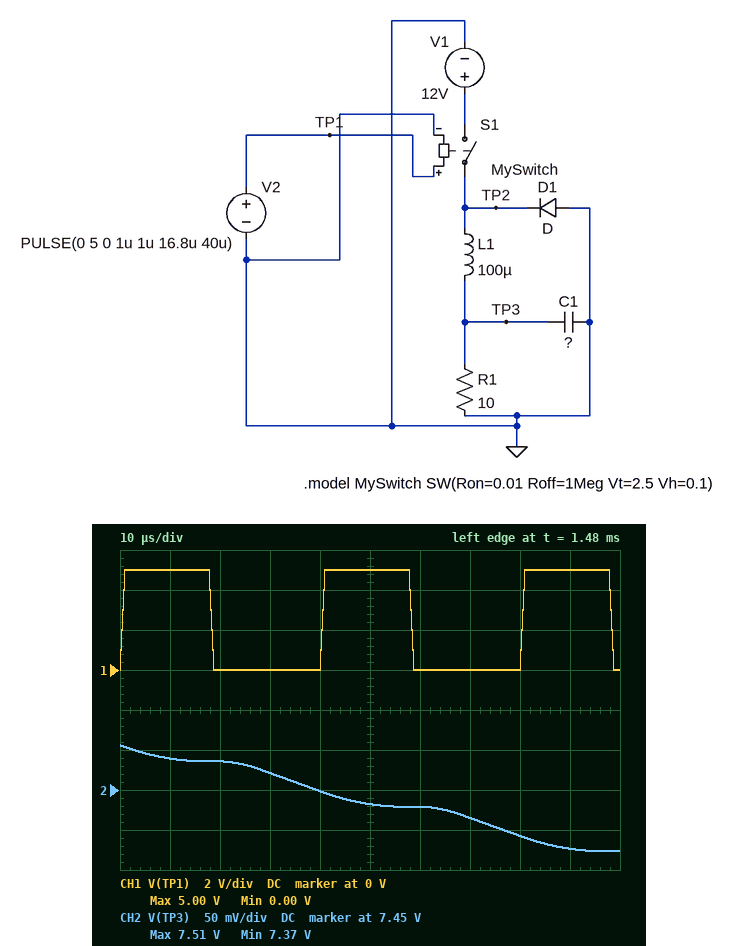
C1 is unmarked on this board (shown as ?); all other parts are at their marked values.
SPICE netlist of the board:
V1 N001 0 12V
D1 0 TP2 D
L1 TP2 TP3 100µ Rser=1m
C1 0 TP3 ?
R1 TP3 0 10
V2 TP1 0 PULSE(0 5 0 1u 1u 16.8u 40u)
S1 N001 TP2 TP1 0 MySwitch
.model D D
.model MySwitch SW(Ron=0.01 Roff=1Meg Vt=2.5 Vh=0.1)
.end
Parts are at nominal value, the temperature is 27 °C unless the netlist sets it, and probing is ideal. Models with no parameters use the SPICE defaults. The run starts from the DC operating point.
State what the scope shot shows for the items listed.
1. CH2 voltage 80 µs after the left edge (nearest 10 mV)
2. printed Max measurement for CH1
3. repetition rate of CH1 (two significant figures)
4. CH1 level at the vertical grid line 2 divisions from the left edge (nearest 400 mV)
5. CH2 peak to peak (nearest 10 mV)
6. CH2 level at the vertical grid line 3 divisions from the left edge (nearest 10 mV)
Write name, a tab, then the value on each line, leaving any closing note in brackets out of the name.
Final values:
CH2 voltage 80 µs after the left edge	7.39 V
printed Max measurement for CH1	5.00 V
repetition rate of CH1	25 kHz
CH1 level at the vertical grid line 2 divisions from the left edge	0 V
CH2 peak to peak	130 mV
CH2 level at the vertical grid line 3 divisions from the left edge	7.47 V
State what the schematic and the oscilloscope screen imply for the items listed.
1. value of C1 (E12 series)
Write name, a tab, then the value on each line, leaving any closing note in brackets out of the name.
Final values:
value of C1	330 µF
